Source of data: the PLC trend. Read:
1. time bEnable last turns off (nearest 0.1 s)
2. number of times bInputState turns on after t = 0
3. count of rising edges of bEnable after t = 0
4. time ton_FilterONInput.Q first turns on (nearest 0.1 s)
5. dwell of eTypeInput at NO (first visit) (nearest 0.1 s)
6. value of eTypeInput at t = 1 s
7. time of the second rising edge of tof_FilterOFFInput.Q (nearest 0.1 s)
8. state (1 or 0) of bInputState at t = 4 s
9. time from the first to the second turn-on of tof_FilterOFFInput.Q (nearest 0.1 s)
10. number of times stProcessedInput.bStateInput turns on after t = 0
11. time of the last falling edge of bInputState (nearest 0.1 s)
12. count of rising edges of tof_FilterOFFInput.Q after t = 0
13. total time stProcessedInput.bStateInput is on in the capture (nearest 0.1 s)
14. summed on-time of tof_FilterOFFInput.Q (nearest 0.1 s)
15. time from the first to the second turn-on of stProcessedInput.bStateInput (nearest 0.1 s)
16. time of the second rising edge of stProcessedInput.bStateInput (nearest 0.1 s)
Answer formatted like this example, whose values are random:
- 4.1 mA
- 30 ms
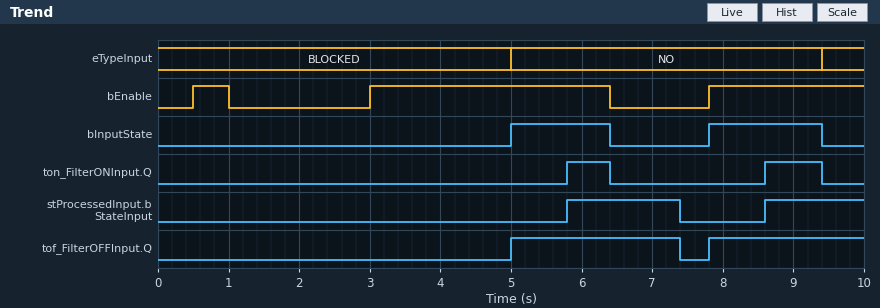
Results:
- 6.4 s
- 2
- 3
- 5.8 s
- 4.4 s
- BLOCKED
- 7.8 s
- 0
- 2.8 s
- 2
- 9.4 s
- 2
- 3.0 s
- 4.6 s
- 2.8 s
- 8.6 s
